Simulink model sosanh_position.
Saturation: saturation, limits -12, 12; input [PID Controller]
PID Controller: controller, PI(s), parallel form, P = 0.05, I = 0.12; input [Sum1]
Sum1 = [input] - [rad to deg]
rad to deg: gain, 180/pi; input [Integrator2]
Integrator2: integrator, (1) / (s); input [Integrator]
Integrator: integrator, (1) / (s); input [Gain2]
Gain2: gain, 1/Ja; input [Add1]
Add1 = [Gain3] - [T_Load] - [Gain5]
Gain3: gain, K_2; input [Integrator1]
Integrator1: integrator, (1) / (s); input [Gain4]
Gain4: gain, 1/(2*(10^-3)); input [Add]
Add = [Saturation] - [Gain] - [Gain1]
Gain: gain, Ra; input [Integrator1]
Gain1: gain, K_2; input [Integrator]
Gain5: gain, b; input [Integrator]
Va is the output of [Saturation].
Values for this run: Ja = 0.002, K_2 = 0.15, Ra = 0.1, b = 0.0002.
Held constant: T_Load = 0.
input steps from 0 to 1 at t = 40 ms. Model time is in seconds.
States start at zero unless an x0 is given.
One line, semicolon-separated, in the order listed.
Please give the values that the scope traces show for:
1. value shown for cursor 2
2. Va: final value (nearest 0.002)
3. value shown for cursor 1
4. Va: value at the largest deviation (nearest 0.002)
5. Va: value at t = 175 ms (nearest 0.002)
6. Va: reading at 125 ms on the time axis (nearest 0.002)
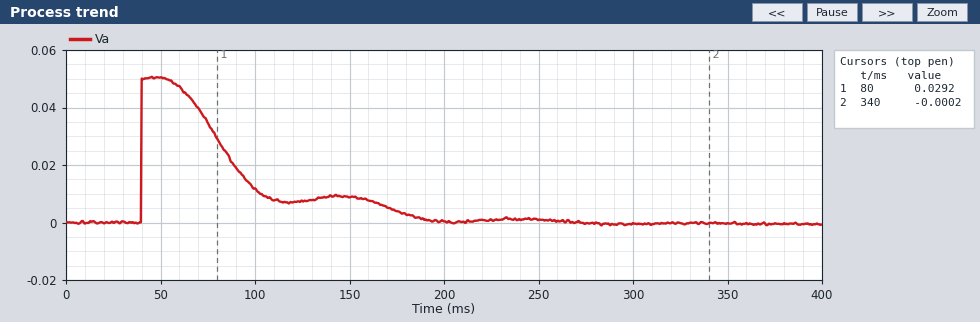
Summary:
-0.0002; 0.000; 0.0292; 0.050; 0.004; 0.008
